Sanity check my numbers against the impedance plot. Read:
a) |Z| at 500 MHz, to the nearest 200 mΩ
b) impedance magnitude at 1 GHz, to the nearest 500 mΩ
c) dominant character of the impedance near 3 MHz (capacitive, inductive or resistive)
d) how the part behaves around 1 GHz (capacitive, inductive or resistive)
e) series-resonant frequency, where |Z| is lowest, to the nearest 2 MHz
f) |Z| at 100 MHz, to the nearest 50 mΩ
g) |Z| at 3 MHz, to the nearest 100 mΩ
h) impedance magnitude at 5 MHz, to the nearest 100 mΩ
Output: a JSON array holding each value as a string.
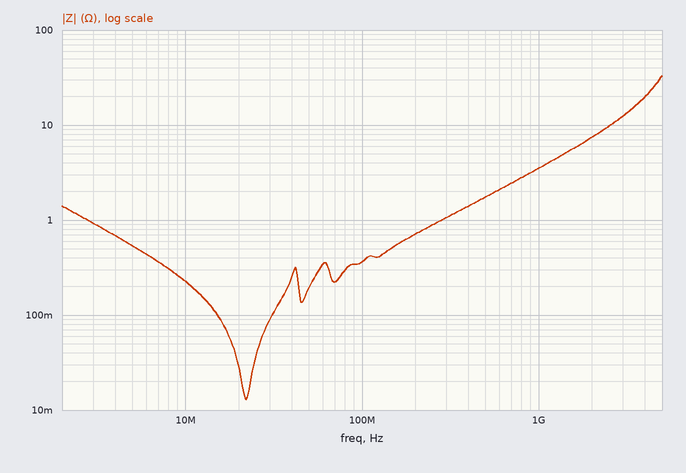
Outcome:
["1.8 Ω", "3.5 Ω", "capacitive", "inductive", "22 MHz", "350 mΩ", "900 mΩ", "500 mΩ"]
